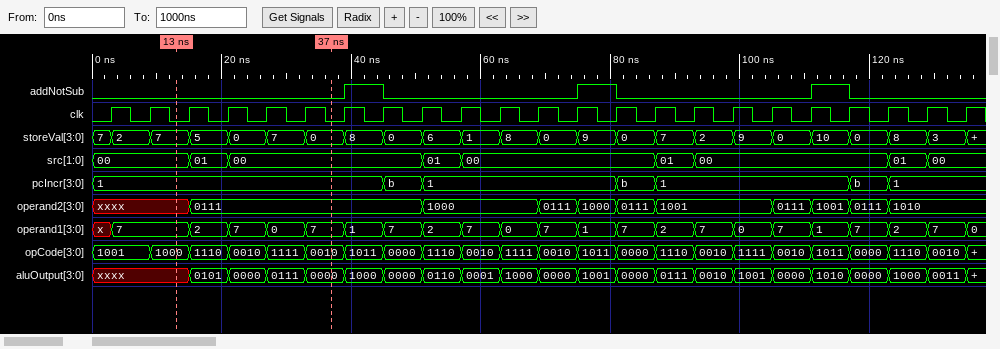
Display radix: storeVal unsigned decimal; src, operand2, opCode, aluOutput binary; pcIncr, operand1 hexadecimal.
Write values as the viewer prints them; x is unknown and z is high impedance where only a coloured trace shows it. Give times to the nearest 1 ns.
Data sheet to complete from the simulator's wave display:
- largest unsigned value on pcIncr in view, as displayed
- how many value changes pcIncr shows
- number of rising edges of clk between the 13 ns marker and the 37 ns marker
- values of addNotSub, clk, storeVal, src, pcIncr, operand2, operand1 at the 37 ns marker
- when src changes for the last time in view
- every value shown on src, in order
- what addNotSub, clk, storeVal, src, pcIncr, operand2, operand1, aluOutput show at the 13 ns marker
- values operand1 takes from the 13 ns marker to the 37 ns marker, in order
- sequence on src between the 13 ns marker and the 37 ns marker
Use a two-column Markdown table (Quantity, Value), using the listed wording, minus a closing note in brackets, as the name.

| Quantity | Value |
|---|---|
| largest unsigned value on pcIncr in view, as displayed | b |
| how many value changes pcIncr shows | 6 |
| number of rising edges of clk between the 13 ns marker and the 37 ns marker | 4 |
| values of addNotSub, clk, storeVal, src, pcIncr, operand2, operand1 at the 37 ns marker | addNotSub=0, clk=0, storeVal=0, src=00, pcIncr=1, operand2=0111, operand1=7 |
| when src changes for the last time in view | 129 ns |
| every value shown on src, in order | 00, 01, 00, 01, 00, 01, 00, 01, 00 |
| what addNotSub, clk, storeVal, src, pcIncr, operand2, operand1, aluOutput show at the 13 ns marker | addNotSub=0, clk=0, storeVal=7, src=00, pcIncr=1, operand2=xxxx, operand1=7, aluOutput=xxxx |
| values operand1 takes from the 13 ns marker to the 37 ns marker, in order | 7, 2, 7, 0, 7 |
| sequence on src between the 13 ns marker and the 37 ns marker | 00, 01, 00 |
